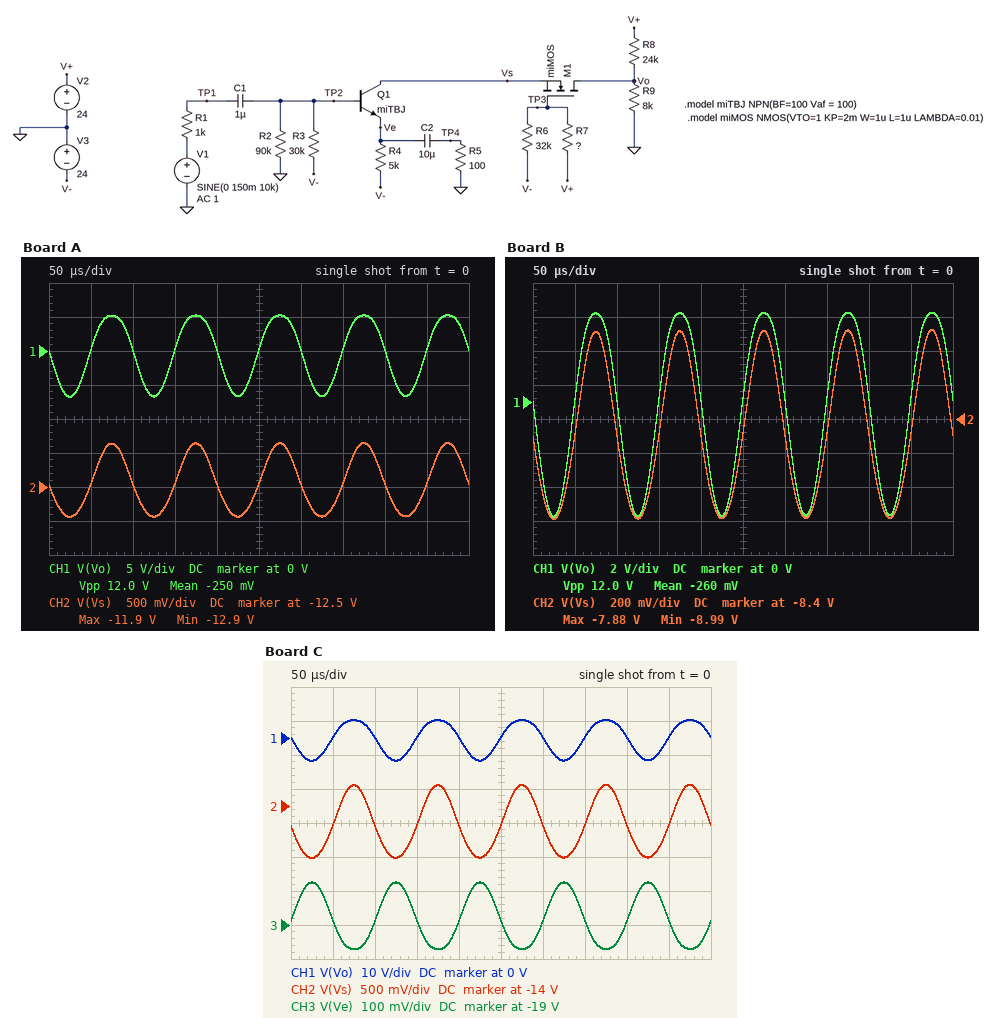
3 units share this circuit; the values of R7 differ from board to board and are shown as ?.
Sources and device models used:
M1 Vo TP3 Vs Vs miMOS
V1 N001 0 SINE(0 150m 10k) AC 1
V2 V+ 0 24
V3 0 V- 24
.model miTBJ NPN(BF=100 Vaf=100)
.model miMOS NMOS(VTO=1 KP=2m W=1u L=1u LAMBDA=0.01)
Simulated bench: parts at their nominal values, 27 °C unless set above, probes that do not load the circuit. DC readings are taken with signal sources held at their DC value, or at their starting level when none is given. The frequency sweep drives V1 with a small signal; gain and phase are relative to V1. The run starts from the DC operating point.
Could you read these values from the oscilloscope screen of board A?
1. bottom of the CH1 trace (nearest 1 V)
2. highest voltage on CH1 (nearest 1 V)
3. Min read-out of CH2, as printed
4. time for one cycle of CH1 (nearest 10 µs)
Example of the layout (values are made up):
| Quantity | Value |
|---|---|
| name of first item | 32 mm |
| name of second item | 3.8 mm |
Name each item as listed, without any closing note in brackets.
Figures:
| Quantity | Value |
|---|---|
| bottom of the CH1 trace | -7 V |
| highest voltage on CH1 | 5 V |
| Min read-out of CH2, as printed | -12.9 V |
| time for one cycle of CH1 | 100 µs |
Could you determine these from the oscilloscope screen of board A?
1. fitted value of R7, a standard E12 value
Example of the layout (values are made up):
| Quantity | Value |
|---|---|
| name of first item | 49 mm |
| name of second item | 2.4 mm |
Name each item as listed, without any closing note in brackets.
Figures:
| Quantity | Value |
|---|---|
| fitted value of R7, a standard E12 value | 82 kΩ |
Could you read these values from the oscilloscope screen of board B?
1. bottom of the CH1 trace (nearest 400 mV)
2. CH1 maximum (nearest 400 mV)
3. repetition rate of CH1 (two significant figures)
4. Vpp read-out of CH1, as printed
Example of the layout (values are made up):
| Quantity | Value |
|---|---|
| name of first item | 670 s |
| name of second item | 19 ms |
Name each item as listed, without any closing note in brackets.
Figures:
| Quantity | Value |
|---|---|
| bottom of the CH1 trace | -6.8 V |
| CH1 maximum | 5.2 V |
| repetition rate of CH1 | 10 kHz |
| Vpp read-out of CH1, as printed | 12.0 V |
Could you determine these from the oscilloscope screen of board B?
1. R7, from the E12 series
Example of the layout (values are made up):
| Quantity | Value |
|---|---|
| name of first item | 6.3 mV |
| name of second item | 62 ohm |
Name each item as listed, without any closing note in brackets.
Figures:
| Quantity | Value |
|---|---|
| R7, from the E12 series | 56 kΩ |
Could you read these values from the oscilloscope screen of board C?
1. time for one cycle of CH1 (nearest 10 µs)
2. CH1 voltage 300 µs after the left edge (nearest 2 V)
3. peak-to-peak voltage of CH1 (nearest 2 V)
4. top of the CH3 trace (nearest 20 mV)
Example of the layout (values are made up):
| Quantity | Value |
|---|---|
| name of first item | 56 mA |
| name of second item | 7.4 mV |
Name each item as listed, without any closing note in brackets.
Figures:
| Quantity | Value |
|---|---|
| time for one cycle of CH1 | 100 µs |
| CH1 voltage 300 µs after the left edge | 0 V |
| peak-to-peak voltage of CH1 | 12 V |
| top of the CH3 trace | -18.88 V |
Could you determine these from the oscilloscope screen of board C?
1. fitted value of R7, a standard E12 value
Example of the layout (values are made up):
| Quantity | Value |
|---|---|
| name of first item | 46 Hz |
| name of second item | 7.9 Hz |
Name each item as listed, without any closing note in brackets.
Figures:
| Quantity | Value |
|---|---|
| fitted value of R7, a standard E12 value | 100 kΩ |
